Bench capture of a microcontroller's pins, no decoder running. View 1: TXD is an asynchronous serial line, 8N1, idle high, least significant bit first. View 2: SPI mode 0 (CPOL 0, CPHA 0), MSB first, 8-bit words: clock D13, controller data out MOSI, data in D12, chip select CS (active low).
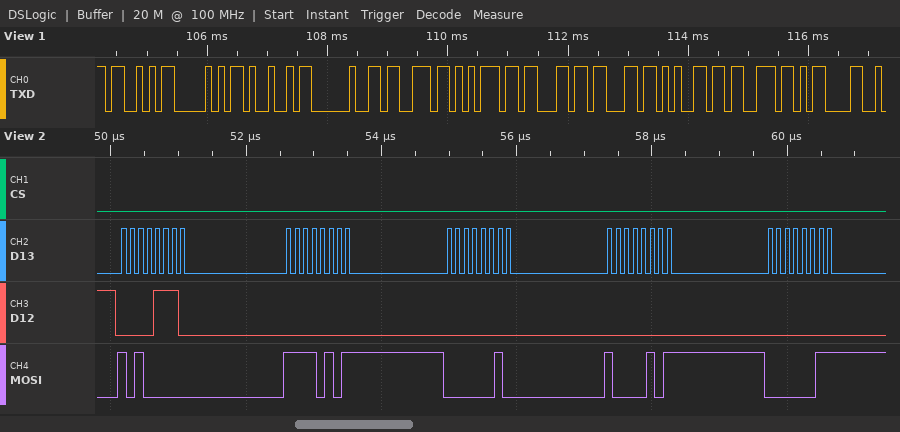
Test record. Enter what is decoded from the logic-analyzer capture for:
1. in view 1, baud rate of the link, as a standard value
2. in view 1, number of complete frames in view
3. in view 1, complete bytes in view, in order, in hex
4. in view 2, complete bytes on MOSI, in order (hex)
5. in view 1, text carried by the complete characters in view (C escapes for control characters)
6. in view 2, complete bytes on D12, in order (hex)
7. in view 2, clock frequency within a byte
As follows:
9600 baud
11
53 50 49 20 73 75 63 63 65 73 0D
A0 F5 02 85 03
"SPI succes\r"
0E 00 00 00 00
8 MHz
